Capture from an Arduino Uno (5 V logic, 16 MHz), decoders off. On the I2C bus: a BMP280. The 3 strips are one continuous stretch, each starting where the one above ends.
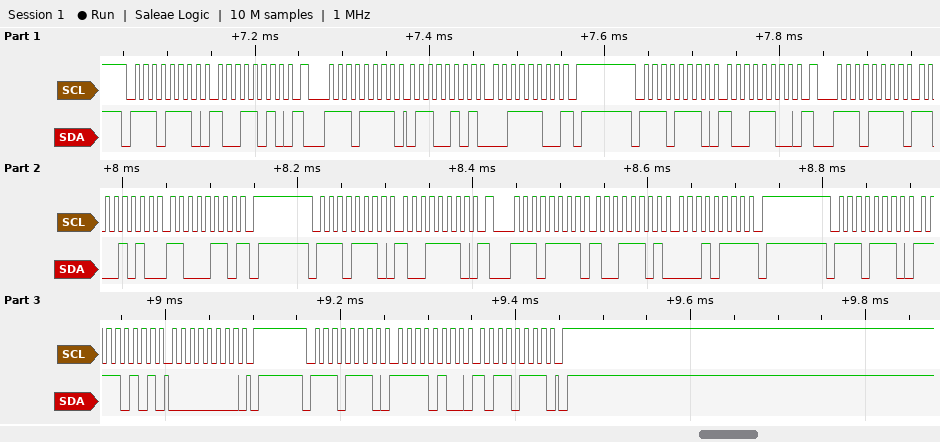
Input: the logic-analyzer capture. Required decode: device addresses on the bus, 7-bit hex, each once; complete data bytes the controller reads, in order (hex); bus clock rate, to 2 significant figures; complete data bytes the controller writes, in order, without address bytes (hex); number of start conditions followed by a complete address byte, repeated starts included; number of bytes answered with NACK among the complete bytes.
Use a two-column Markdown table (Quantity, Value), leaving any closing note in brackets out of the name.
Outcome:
| Quantity | Value |
|---|---|
| device addresses on the bus, 7-bit hex, each once | 0x77 |
| complete data bytes the controller reads, in order | 65 3C CA C6 9D 17 |
| bus clock rate, to 2 significant figures | 100 kHz |
| complete data bytes the controller writes, in order, without address bytes | 9A 9C 9E F5 00 F4 B7 |
| number of start conditions followed by a complete address byte, repeated starts included | 8 |
| number of bytes answered with NACK among the complete bytes | 3 |
